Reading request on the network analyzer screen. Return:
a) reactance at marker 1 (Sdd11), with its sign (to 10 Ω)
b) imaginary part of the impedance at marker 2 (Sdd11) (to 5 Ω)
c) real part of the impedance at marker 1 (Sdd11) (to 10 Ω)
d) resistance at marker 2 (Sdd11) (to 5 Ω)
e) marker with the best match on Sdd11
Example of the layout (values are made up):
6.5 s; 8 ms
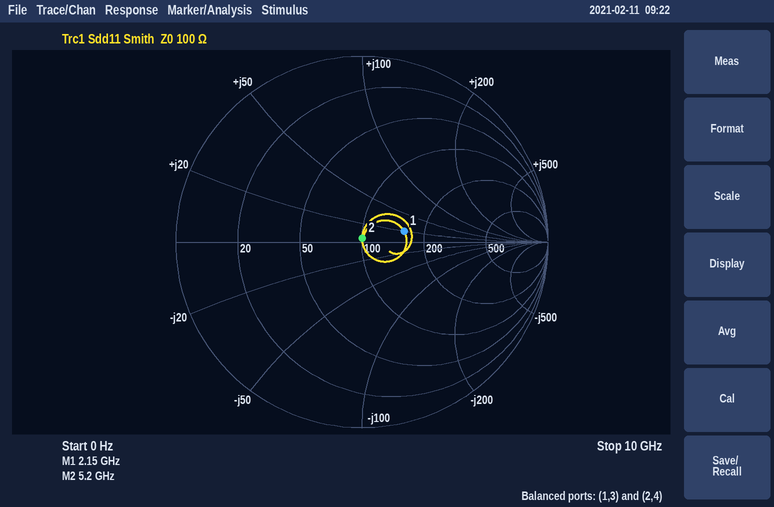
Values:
+20 Ω; +5 Ω; 160 Ω; 100 Ω; marker 2
